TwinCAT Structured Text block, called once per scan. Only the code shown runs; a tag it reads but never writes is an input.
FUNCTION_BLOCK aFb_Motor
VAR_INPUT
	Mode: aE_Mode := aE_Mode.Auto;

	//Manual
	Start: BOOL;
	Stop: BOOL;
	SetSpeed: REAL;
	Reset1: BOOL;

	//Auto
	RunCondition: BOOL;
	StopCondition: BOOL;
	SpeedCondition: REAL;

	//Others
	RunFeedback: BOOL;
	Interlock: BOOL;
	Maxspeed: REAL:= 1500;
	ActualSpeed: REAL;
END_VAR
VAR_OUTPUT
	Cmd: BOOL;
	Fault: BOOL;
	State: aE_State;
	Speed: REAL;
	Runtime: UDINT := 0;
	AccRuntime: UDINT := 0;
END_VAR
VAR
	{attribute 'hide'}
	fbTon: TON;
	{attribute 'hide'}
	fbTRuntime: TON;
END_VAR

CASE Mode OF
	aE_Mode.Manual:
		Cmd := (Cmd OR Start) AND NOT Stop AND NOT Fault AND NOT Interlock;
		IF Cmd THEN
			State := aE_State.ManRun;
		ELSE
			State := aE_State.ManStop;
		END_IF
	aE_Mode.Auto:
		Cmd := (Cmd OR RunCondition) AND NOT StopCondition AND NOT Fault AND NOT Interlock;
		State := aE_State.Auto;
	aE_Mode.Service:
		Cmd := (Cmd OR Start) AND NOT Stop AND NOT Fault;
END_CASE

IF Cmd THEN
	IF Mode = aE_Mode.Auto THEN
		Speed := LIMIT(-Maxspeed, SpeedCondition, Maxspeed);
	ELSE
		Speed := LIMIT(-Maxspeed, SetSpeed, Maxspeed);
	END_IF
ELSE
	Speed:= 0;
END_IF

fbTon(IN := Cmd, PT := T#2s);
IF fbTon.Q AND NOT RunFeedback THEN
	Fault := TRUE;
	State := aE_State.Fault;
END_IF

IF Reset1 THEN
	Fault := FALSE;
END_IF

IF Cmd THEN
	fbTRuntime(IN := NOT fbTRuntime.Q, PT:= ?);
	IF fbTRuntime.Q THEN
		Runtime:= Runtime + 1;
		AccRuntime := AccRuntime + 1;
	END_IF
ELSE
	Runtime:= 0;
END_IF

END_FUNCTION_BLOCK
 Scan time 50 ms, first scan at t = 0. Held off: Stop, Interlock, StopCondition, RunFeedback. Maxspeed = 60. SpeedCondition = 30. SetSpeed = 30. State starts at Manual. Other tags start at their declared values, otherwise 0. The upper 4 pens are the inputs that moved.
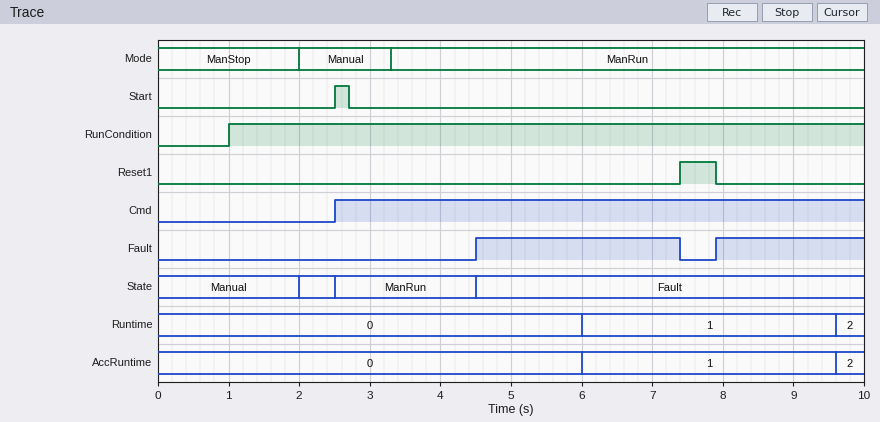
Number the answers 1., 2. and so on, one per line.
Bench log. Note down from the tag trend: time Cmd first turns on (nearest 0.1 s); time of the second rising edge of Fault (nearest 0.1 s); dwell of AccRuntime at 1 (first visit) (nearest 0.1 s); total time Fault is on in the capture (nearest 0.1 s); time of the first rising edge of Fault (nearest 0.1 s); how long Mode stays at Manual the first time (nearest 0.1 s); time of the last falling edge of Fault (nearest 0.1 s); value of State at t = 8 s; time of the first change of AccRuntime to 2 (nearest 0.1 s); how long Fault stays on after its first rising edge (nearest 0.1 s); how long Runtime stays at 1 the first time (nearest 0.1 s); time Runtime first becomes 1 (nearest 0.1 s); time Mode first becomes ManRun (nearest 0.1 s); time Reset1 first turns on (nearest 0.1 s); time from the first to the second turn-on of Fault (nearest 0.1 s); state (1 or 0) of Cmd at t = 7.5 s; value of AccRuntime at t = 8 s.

1. 2.5 s
2. 7.9 s
3. 3.6 s
4. 5.0 s
5. 4.5 s
6. 1.3 s
7. 7.4 s
8. Fault
9. 9.6 s
10. 2.9 s
11. 3.6 s
12. 6.0 s
13. 3.3 s
14. 7.4 s
15. 3.4 s
16. 1
17. 1
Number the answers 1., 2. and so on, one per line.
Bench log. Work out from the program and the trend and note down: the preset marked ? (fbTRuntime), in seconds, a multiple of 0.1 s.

1. 3.5 s
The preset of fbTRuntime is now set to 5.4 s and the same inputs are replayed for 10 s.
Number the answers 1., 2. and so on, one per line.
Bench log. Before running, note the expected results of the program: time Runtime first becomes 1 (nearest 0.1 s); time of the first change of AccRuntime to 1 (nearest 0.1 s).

1. 7.9 s
2. 7.9 s
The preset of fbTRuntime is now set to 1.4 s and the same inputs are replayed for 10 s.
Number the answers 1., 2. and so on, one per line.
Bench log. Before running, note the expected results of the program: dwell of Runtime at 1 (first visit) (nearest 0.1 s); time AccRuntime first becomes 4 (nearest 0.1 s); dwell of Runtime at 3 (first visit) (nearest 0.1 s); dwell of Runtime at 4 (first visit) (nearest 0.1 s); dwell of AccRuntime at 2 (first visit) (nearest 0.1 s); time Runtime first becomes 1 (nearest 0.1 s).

1. 1.5 s
2. 8.4 s
3. 1.5 s
4. 1.5 s
5. 1.5 s
6. 3.9 s
